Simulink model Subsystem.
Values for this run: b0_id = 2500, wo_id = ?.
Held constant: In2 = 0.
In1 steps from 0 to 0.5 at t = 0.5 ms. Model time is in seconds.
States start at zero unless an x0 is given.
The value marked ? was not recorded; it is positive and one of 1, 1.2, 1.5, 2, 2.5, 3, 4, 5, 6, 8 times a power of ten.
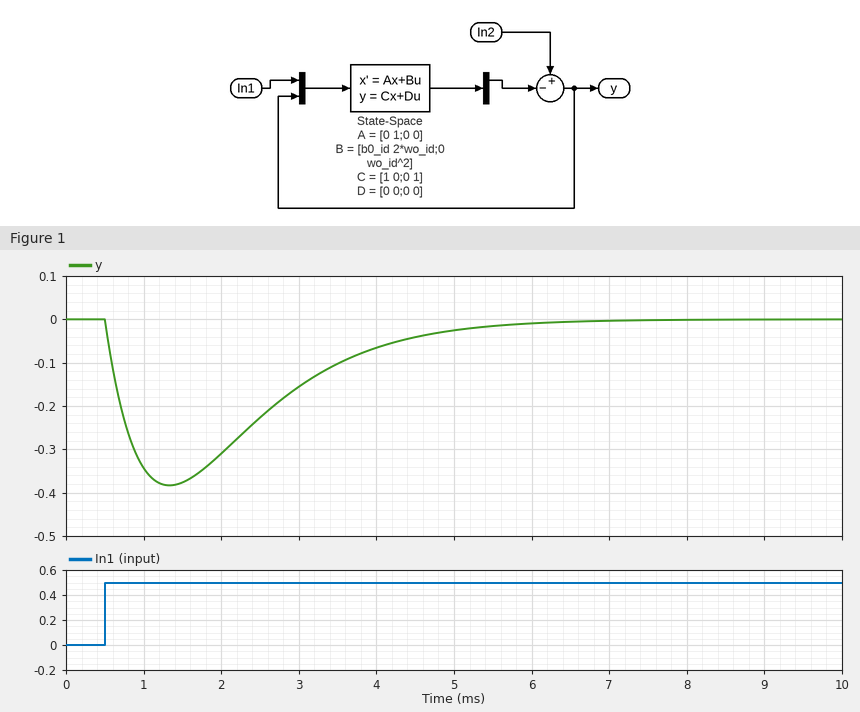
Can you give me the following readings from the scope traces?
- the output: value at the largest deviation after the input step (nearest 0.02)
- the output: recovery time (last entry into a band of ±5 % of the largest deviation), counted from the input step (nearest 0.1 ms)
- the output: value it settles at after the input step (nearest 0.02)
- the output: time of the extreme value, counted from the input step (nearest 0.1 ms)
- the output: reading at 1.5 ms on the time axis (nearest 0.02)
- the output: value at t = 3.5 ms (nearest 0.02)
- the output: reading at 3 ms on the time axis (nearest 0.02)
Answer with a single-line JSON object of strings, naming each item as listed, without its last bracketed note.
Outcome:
{"the output: value at the largest deviation after the input step": "-0.38", "the output: recovery time (last entry into a band of ±5 % of the largest deviation), counted from the input step": "4.8 ms", "the output: value it settles at after the input step": "0.00", "the output: time of the extreme value, counted from the input step": "0.8 ms", "the output: reading at 1.5 ms on the time axis": "-0.38", "the output: value at t = 3.5 ms": "-0.10", "the output: reading at 3 ms on the time axis": "-0.16"}
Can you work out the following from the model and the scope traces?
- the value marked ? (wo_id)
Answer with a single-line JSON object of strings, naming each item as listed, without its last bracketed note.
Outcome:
{"the value marked ?": "1200"}
